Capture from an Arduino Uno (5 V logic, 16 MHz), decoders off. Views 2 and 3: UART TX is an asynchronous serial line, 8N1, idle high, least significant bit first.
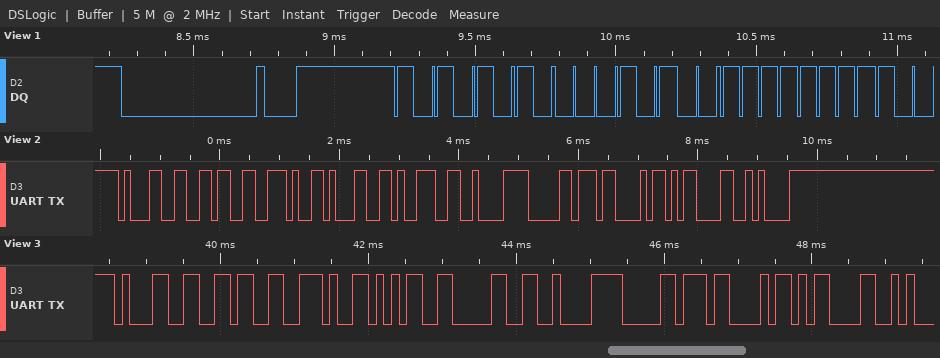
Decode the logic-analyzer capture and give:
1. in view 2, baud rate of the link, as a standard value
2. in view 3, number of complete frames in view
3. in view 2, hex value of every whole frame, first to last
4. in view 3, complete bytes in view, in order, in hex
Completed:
9600 baud
9
0x31 0x36 0x2E 0x31 0x39 0xC2 0xB0 0x43 0x0D 0x0A
0x31 0x36 0x2E 0x35 0x30 0xC2 0xB0 0x43 0x0D
